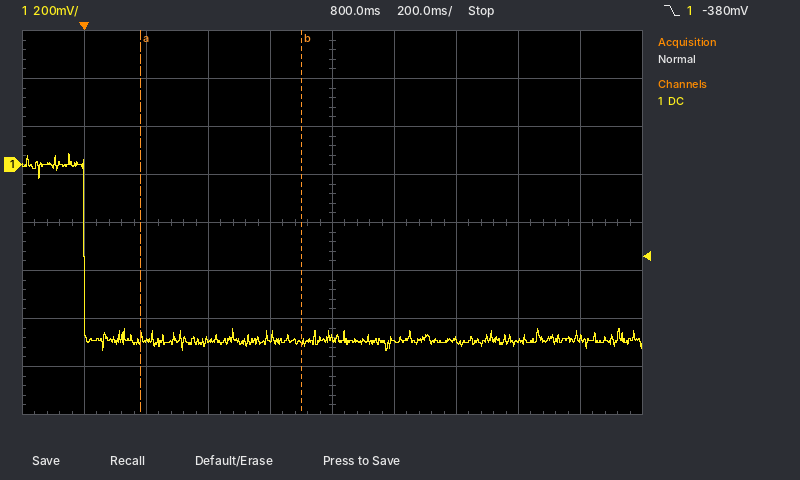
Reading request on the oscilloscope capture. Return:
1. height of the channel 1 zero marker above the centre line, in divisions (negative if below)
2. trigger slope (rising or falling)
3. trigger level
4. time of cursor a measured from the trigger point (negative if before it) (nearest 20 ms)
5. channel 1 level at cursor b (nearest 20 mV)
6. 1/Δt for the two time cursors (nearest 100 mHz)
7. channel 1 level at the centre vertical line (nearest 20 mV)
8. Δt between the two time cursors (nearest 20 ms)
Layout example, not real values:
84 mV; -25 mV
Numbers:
+1.2 div; falling; -380 mV; +180 ms; -740 mV; 1.9 Hz; -720 mV; 520 ms
